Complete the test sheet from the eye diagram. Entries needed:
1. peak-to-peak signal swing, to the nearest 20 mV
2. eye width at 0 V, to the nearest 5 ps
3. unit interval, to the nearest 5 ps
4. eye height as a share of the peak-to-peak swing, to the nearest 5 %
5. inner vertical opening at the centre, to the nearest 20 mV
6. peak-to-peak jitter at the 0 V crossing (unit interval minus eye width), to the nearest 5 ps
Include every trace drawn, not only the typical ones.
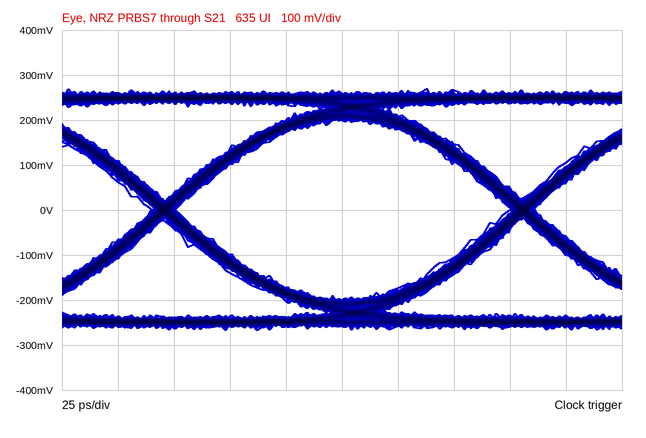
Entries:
540 mV
150 ps
160 ps
75 %
400 mV
10 ps
